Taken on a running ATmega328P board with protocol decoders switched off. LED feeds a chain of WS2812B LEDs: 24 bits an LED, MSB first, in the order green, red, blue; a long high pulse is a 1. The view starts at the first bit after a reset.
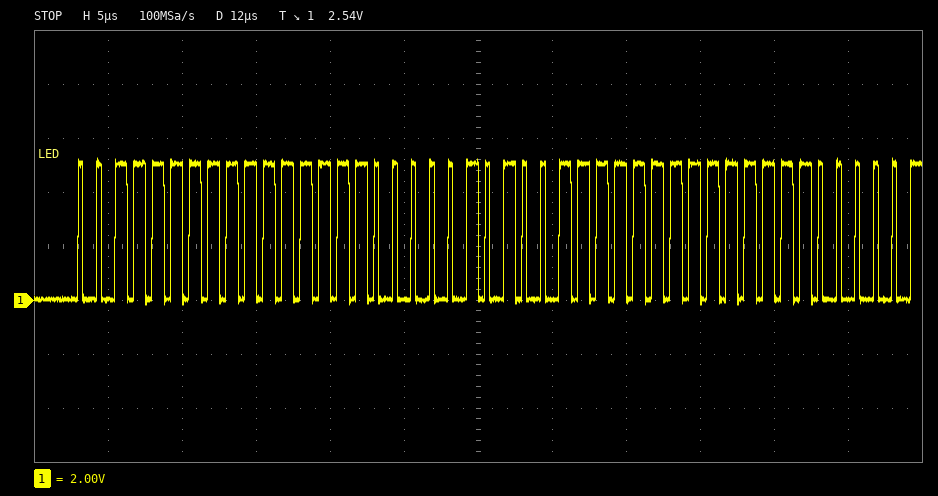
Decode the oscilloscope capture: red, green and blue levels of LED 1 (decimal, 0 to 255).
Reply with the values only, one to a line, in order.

255, 63, 5
